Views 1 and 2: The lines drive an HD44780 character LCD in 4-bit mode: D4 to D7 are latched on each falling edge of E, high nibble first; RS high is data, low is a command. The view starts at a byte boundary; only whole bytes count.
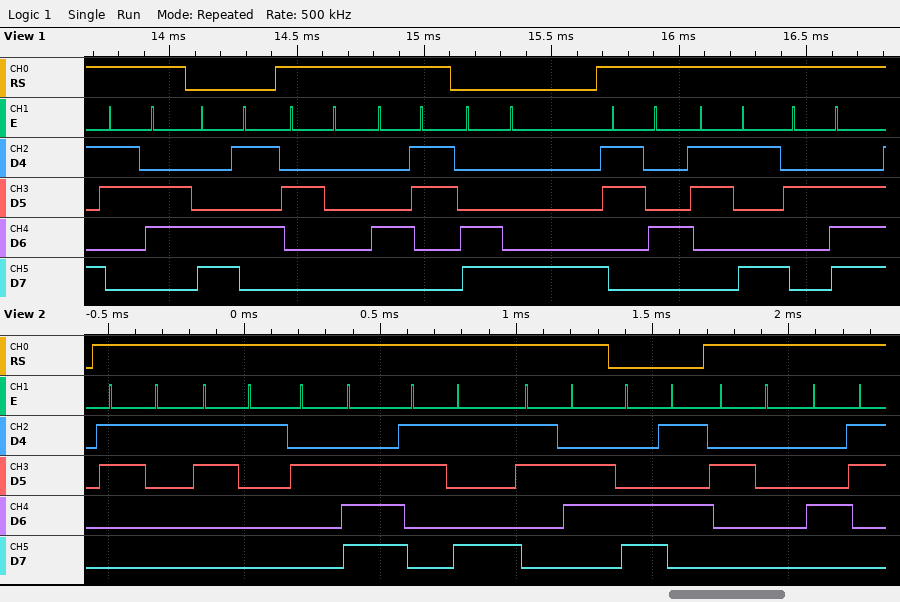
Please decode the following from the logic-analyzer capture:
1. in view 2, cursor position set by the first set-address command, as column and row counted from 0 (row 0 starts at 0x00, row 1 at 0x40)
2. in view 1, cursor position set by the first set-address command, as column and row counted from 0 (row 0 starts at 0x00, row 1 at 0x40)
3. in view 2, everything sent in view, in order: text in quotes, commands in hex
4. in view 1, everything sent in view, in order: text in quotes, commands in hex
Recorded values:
column 5, row 1
column 5, row 1
"11.96" 0xC5 " C"
"6" 0xC5 " C" 0xC8 "49."
